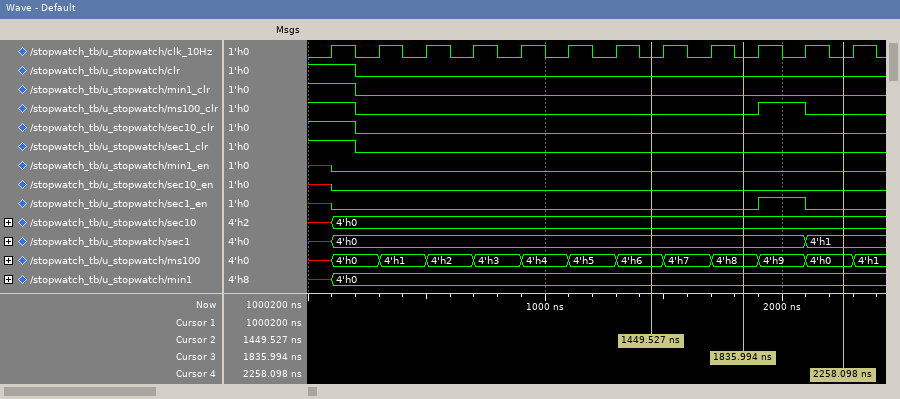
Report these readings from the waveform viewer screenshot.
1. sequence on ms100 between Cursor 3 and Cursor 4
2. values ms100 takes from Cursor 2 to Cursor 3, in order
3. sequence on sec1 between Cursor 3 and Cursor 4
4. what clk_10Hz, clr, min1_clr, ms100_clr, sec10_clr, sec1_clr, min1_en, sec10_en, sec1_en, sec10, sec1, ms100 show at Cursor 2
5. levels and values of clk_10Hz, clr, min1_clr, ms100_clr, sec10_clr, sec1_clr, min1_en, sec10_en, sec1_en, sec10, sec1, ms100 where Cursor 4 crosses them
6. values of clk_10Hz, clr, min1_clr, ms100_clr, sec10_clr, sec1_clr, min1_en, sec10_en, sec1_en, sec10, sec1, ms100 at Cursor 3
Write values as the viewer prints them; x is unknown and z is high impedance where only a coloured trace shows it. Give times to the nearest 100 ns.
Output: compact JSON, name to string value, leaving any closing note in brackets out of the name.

{"sequence on ms100 between Cursor 3 and Cursor 4": "4'h8, 4'h9, 4'h0", "values ms100 takes from Cursor 2 to Cursor 3, in order": "4'h6, 4'h7, 4'h8", "sequence on sec1 between Cursor 3 and Cursor 4": "4'h0, 4'h1", "what clk_10Hz, clr, min1_clr, ms100_clr, sec10_clr, sec1_clr, min1_en, sec10_en, sec1_en, sec10, sec1, ms100 show at Cursor 2": "clk_10Hz=0, clr=0, min1_clr=0, ms100_clr=0, sec10_clr=0, sec1_clr=0, min1_en=0, sec10_en=0, sec1_en=0, sec10=4'h0, sec1=4'h0, ms100=4'h6", "levels and values of clk_10Hz, clr, min1_clr, ms100_clr, sec10_clr, sec1_clr, min1_en, sec10_en, sec1_en, sec10, sec1, ms100 where Cursor 4 crosses them": "clk_10Hz=0, clr=0, min1_clr=0, ms100_clr=0, sec10_clr=0, sec1_clr=0, min1_en=0, sec10_en=0, sec1_en=0, sec10=4'h0, sec1=4'h1, ms100=4'h0", "values of clk_10Hz, clr, min1_clr, ms100_clr, sec10_clr, sec1_clr, min1_en, sec10_en, sec1_en, sec10, sec1, ms100 at Cursor 3": "clk_10Hz=0, clr=0, min1_clr=0, ms100_clr=0, sec10_clr=0, sec1_clr=0, min1_en=0, sec10_en=0, sec1_en=0, sec10=4'h0, sec1=4'h0, ms100=4'h8"}
